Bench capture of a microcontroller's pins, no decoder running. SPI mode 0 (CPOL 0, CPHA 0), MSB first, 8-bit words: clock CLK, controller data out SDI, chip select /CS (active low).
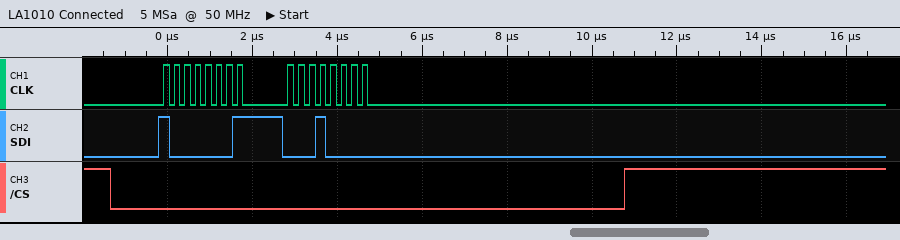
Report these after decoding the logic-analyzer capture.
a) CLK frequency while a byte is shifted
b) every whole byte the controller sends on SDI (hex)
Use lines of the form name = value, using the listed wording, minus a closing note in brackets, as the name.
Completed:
CLK frequency while a byte is shifted = 4 MHz
every whole byte the controller sends on SDI = 0x81 0x10
